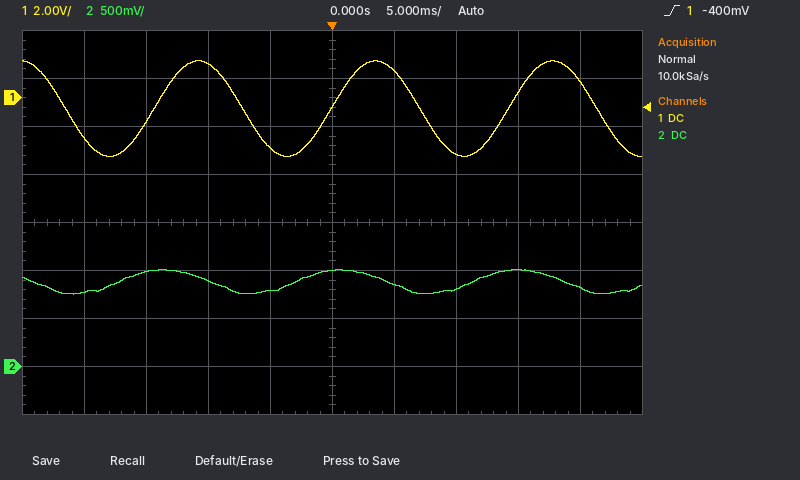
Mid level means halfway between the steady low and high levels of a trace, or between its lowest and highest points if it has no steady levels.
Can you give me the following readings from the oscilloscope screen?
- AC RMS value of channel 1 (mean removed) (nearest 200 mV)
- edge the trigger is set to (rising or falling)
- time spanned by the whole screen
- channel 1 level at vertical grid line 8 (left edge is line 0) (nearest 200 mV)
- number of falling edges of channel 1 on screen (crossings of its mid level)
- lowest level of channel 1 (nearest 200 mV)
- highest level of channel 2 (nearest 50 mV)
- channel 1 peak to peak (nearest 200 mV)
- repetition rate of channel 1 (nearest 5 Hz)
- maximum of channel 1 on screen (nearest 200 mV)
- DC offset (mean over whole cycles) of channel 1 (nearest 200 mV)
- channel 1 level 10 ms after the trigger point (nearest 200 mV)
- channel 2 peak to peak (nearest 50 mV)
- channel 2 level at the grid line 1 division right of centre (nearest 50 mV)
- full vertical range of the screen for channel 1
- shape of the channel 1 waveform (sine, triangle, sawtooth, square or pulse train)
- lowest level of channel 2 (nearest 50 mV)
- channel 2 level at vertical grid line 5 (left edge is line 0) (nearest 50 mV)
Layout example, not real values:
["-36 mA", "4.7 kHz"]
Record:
["1.4 V", "rising", "50 ms", "200 mV", "4", "-2.4 V", "1.00 V", "4.0 V", "70 Hz", "1.6 V", "-400 mV", "-2.4 V", "250 mV", "850 mV", "16 V", "sine", "750 mV", "1.00 V"]
